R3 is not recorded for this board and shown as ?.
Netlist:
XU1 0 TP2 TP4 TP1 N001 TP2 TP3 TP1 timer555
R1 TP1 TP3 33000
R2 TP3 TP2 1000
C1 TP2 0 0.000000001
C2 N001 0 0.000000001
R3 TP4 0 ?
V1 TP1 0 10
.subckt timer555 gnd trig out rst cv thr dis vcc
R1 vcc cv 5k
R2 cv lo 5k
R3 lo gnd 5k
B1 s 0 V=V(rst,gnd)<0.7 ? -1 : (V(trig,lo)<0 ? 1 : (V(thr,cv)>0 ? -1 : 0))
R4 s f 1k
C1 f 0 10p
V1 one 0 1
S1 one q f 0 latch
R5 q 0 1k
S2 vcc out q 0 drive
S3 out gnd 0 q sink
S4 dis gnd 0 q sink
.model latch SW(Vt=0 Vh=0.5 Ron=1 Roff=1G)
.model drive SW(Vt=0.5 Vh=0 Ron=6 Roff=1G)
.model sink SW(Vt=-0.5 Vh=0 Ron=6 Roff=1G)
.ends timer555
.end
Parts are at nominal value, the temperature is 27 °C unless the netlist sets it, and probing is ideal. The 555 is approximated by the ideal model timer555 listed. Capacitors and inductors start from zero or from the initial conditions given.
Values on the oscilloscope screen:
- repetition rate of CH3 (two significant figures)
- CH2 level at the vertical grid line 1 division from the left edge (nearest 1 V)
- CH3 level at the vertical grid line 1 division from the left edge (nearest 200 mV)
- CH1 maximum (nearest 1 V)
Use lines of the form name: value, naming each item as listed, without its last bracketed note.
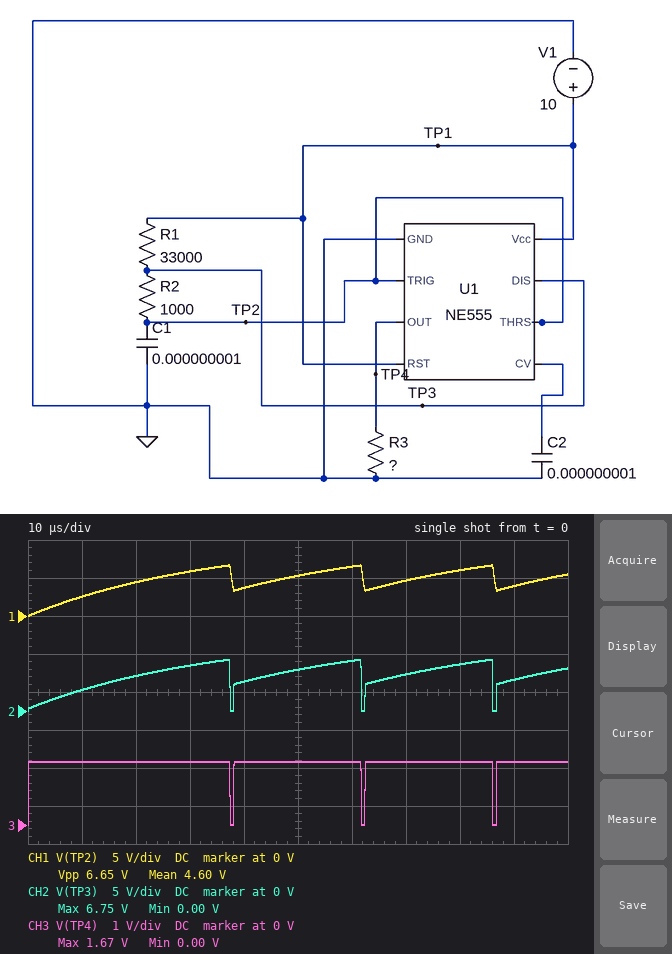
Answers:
repetition rate of CH3: 41 kHz
CH2 level at the vertical grid line 1 division from the left edge: 3 V
CH3 level at the vertical grid line 1 division from the left edge: 1.6 V
CH1 maximum: 7 V
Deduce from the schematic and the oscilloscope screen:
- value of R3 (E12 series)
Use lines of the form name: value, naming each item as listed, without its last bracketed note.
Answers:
value of R3: 1.2 Ω
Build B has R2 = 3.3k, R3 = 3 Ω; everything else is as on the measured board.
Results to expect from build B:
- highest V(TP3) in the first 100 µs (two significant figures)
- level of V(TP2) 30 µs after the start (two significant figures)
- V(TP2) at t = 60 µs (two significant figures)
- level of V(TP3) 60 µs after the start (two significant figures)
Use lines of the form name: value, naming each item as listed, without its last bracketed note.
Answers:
highest V(TP3) in the first 100 µs: 7.0 V
level of V(TP2) 30 µs after the start: 5.6 V
V(TP2) at t = 60 µs: 5.9 V
level of V(TP3) 60 µs after the start: 6.3 V
